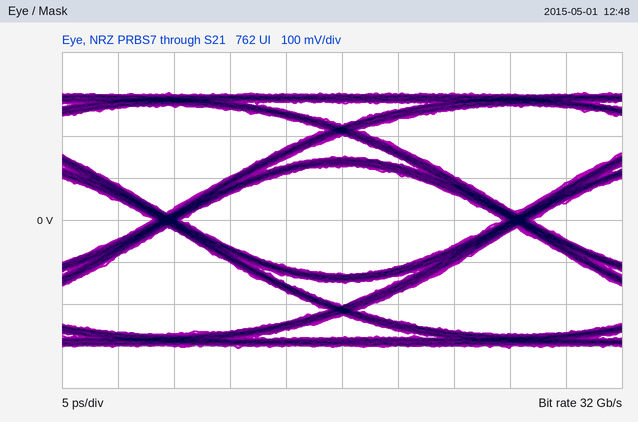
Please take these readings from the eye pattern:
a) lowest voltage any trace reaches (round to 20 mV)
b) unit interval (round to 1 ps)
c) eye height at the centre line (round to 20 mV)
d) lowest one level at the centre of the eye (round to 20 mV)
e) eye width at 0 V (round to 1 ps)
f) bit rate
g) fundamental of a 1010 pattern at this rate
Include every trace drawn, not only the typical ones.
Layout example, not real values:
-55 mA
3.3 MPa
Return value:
-300 mV
31 ps
260 mV
120 mV
29 ps
32 Gb/s
16 GHz
